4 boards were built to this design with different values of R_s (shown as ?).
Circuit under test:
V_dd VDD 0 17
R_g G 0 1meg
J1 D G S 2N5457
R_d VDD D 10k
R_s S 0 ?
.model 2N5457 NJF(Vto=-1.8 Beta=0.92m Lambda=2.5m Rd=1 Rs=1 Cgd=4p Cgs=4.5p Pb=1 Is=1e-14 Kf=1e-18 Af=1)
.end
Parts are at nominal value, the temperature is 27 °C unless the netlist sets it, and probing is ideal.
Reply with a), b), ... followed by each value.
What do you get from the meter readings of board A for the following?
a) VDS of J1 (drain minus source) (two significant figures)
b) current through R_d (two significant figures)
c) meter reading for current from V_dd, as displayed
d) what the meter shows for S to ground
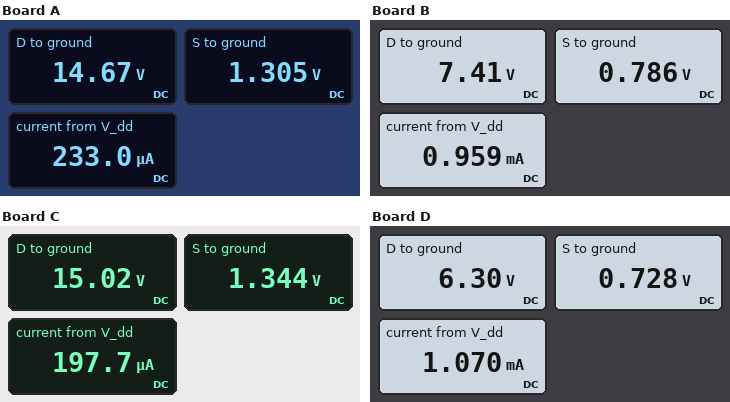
a) 13 V
b) 230 µA
c) 233.0 µA
d) 1.305 V
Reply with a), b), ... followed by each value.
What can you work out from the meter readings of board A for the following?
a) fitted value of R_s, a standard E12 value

a) 5.6 kΩ
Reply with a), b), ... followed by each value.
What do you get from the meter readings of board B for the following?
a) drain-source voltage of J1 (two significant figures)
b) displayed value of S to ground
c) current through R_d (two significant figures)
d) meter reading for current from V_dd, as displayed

a) 6.6 V
b) 0.786 V
c) 960 µA
d) 0.959 mA
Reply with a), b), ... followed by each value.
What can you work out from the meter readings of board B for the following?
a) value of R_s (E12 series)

a) 820 Ω
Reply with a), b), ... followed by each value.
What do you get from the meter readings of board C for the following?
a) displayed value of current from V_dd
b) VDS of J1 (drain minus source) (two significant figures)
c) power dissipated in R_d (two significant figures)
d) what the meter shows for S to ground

a) 197.7 µA
b) 14 V
c) 390 µW
d) 1.344 V
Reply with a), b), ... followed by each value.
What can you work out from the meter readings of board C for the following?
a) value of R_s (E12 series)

a) 6.8 kΩ
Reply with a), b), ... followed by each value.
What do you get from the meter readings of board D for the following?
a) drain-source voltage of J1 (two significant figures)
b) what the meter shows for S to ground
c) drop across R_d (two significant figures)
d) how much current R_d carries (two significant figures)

a) 5.6 V
b) 0.728 V
c) 11 V
d) 1.1 mA
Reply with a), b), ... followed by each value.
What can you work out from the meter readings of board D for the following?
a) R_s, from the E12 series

a) 680 Ω
